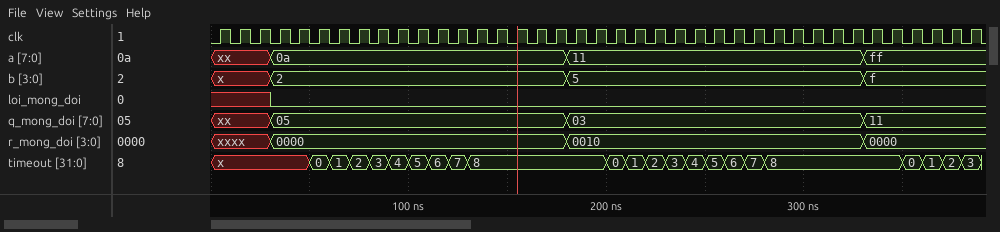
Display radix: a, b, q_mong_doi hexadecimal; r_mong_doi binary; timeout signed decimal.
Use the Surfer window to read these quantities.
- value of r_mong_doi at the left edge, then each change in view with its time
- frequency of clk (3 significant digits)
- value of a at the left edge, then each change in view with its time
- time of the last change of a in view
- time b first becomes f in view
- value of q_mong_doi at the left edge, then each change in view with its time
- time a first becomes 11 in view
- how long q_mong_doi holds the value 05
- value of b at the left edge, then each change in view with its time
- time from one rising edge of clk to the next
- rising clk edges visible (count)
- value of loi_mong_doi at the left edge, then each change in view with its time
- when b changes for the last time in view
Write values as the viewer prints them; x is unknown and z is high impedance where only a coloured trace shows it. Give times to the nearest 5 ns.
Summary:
xxxx, 0000 at 30 ns, 0010 at 180 ns, 0000 at 330 ns
100 MHz
xx, 0a at 30 ns, 11 at 180 ns, ff at 330 ns
330 ns
330 ns
xx, 05 at 30 ns, 03 at 180 ns, 11 at 330 ns
180 ns
150 ns
x, 2 at 30 ns, 5 at 180 ns, f at 330 ns
10 ns
39
x, 0 at 30 ns
330 ns
